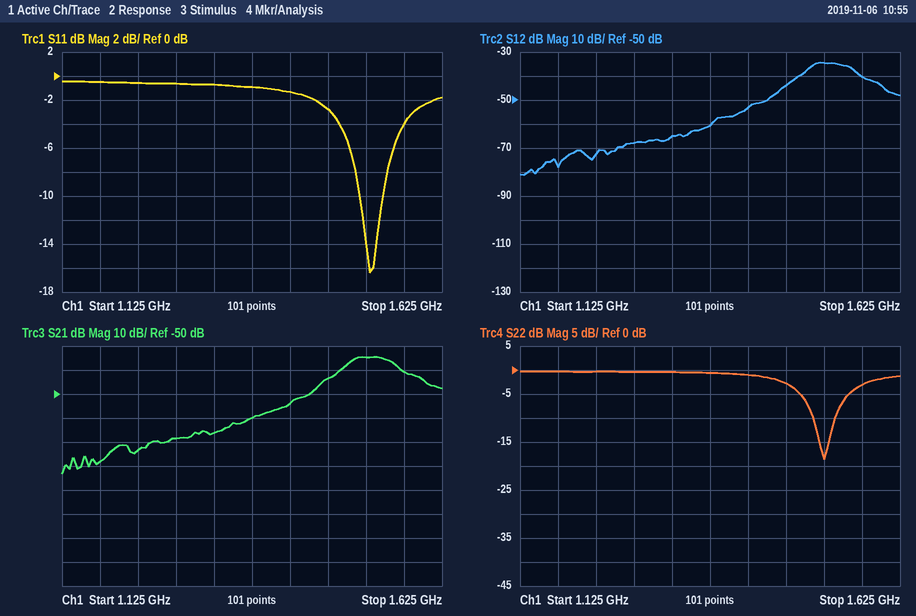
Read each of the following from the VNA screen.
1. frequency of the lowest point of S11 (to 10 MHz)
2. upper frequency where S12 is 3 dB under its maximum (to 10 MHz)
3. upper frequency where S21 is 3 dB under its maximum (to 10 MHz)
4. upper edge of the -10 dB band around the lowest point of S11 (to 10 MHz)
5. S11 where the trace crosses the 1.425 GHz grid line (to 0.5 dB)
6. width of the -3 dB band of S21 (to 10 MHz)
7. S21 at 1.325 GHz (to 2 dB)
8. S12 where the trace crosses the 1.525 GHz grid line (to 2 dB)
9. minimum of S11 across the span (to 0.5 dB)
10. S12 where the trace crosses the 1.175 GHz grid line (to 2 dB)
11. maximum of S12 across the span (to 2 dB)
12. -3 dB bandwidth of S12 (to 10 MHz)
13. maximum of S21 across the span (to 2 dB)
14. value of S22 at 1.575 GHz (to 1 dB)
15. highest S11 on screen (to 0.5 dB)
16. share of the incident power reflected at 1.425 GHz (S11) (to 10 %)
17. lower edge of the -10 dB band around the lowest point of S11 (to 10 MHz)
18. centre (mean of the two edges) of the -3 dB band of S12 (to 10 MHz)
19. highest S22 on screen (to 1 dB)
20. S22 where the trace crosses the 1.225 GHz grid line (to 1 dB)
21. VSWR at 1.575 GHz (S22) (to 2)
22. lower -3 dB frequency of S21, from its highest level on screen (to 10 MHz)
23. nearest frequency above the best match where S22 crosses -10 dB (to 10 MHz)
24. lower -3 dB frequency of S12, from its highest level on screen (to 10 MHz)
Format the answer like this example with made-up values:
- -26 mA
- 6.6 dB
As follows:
- 1.53 GHz
- 1.56 GHz
- 1.56 GHz
- 1.55 GHz
- -1.5 dB
- 60 MHz
- -66 dB
- -34 dB
- -16.5 dB
- -78 dB
- -34 dB
- 60 MHz
- -34 dB
- -3 dB
- -0.5 dB
- 70 %
- 1.52 GHz
- 1.53 GHz
- 0 dB
- 0 dB
- 6
- 1.50 GHz
- 1.54 GHz
- 1.50 GHz
